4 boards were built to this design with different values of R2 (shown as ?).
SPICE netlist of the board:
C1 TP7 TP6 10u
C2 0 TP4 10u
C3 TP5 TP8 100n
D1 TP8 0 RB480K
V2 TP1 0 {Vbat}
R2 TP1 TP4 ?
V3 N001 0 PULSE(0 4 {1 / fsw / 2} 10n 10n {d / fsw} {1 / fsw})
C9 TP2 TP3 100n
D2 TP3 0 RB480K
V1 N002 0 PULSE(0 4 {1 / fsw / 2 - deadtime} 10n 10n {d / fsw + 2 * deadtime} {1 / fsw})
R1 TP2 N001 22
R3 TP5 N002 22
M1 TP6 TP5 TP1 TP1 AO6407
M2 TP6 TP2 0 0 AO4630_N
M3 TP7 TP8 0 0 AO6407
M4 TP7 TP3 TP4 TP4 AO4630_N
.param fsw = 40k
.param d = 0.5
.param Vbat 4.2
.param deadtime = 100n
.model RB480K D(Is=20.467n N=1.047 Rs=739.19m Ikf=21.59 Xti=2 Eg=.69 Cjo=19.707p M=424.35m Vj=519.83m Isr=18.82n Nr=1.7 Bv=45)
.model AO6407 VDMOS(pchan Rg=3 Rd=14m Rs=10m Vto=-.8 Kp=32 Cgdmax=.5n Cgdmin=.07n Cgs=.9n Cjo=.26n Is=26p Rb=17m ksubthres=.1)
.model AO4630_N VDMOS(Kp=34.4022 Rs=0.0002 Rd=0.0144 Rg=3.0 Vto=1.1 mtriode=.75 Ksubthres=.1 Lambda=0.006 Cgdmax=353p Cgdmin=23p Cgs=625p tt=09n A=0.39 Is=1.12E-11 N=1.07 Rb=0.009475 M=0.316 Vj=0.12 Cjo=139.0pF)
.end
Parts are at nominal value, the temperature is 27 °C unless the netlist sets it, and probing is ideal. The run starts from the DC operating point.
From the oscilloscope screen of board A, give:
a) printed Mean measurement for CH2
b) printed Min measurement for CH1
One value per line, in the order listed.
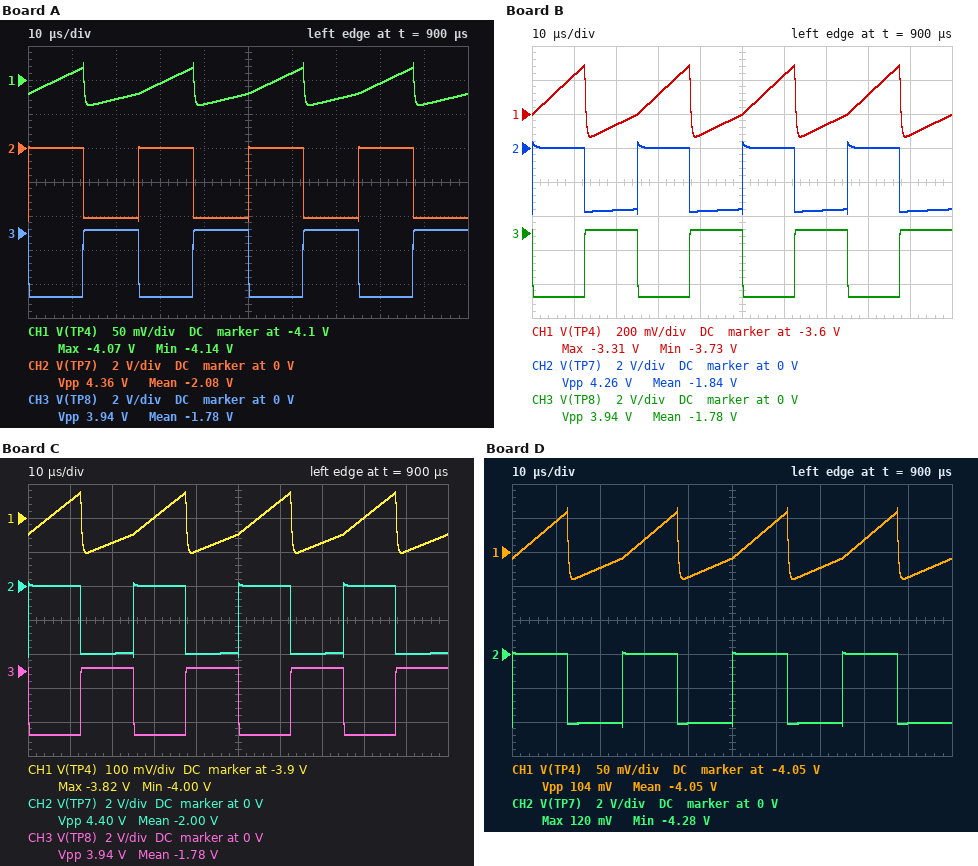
-2.08 V
-4.14 V
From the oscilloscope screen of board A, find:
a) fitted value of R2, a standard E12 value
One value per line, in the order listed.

270 Ω
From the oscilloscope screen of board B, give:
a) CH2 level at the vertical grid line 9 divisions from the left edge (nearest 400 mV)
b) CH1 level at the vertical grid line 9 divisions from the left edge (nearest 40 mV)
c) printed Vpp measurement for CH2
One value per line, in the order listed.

-3.6 V
-3.72 V
4.26 V
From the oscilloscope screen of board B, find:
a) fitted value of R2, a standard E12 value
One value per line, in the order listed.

33 Ω
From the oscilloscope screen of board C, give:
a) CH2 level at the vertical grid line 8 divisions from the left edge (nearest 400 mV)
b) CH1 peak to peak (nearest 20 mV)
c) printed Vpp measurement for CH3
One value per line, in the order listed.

0 V
180 mV
3.94 V
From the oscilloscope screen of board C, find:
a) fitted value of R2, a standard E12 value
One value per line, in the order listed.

82 Ω
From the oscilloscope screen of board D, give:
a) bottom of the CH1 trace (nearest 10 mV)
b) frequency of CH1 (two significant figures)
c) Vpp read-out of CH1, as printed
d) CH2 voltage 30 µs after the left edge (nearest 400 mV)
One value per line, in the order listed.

-4.09 V
40 kHz
104 mV
0 V
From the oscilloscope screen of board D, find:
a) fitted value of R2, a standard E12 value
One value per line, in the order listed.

150 Ω
